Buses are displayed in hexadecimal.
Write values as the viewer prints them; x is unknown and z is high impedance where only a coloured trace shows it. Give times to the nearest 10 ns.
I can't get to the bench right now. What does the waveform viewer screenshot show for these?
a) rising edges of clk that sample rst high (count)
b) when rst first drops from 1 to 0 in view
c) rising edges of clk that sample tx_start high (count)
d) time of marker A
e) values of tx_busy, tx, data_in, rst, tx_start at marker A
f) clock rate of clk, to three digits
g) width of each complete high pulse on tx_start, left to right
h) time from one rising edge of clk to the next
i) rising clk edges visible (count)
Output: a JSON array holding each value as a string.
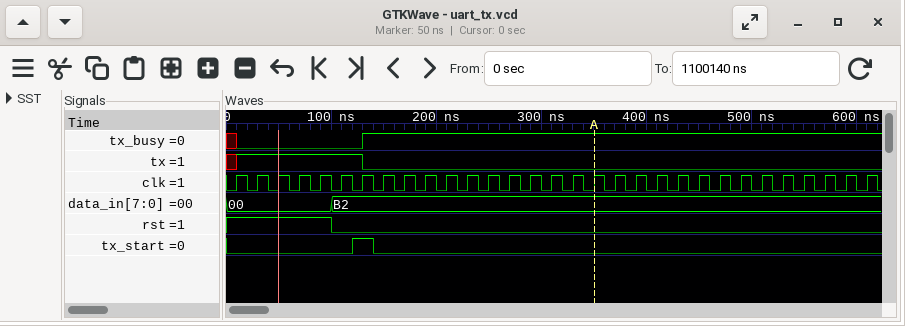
["5", "100 ns", "1", "350 ns", "tx_busy=1, tx=0, data_in=B2, rst=0, tx_start=0", "50.0 MHz", "20 ns", "20 ns", "31"]
